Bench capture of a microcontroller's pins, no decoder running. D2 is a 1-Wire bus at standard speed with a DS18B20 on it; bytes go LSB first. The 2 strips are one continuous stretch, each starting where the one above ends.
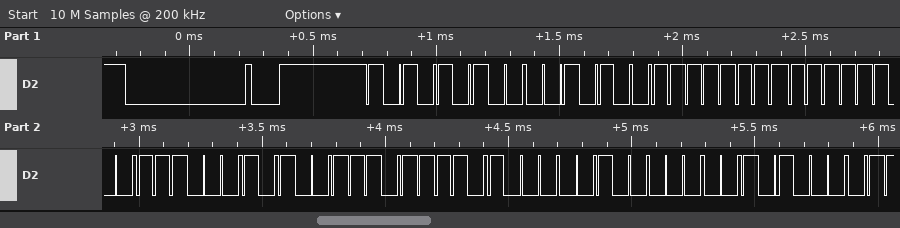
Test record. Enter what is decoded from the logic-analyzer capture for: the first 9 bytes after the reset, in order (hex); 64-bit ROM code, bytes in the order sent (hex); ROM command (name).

55 28 FF 3F 47 B9 17 04 14
28 FF 3F 47 B9 17 04 14
Match ROM
